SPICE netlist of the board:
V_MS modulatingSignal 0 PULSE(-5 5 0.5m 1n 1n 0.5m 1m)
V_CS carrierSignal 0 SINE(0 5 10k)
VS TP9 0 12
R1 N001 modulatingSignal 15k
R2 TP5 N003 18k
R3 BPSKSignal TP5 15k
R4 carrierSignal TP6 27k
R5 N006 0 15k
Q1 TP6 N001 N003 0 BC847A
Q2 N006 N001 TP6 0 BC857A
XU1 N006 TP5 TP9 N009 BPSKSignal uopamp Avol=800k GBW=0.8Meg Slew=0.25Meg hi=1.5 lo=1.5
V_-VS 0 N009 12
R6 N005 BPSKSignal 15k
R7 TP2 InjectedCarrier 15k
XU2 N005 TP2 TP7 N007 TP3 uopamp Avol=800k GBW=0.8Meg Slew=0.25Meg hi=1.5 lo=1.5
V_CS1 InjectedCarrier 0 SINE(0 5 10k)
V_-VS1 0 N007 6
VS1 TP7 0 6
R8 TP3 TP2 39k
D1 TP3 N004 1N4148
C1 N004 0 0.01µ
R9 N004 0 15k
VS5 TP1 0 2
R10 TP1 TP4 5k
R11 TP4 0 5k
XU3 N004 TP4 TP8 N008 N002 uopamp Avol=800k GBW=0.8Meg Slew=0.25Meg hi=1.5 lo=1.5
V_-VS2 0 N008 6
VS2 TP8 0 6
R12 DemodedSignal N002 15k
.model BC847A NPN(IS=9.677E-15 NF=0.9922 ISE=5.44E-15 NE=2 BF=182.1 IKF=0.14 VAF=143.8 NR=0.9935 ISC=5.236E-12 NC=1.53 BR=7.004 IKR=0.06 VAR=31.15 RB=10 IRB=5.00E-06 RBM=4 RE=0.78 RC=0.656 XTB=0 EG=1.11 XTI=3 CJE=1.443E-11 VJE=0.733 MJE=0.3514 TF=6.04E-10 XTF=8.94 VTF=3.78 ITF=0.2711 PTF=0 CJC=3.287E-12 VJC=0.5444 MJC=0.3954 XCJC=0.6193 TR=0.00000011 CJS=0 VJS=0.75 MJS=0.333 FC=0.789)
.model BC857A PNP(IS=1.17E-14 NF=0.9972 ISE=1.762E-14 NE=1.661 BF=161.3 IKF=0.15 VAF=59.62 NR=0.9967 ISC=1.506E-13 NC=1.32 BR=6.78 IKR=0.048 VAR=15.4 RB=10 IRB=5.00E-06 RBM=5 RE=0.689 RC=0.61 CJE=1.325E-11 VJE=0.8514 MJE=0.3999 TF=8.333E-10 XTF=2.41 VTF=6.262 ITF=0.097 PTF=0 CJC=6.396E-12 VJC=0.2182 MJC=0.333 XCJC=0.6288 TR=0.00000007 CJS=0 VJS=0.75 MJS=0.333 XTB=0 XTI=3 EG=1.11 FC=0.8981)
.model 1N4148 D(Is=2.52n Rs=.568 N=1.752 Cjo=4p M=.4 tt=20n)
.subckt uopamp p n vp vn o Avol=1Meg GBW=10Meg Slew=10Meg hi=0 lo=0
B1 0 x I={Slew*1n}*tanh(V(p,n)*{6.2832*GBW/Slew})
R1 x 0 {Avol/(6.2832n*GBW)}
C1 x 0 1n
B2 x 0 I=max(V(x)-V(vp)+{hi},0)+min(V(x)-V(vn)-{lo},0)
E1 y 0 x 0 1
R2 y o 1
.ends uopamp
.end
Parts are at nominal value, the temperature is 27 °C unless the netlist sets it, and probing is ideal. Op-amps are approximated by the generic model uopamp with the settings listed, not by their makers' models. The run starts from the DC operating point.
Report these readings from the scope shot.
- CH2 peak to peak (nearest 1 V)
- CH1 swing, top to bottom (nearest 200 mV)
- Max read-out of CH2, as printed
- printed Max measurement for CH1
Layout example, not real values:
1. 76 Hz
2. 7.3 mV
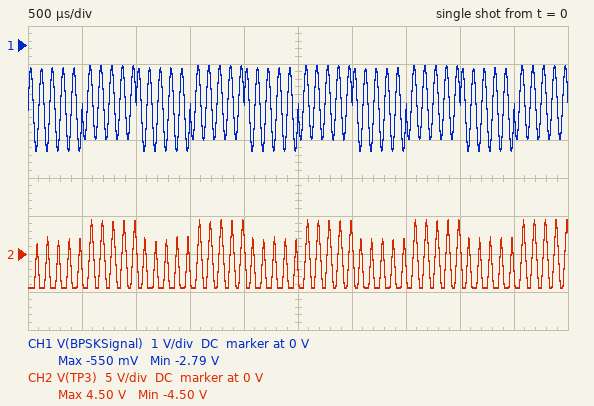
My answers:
1. 9 V
2. 2.2 V
3. 4.50 V
4. -550 mV
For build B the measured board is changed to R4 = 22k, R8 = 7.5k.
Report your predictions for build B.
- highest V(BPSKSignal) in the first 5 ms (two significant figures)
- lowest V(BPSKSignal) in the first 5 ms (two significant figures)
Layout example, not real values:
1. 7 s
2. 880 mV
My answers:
1. -310 mV
2. -2.9 V
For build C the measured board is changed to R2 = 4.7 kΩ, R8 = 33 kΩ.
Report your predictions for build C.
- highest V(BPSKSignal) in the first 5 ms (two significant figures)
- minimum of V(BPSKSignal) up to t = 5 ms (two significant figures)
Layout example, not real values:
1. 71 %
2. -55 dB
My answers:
1. -610 mV
2. -4.8 V
